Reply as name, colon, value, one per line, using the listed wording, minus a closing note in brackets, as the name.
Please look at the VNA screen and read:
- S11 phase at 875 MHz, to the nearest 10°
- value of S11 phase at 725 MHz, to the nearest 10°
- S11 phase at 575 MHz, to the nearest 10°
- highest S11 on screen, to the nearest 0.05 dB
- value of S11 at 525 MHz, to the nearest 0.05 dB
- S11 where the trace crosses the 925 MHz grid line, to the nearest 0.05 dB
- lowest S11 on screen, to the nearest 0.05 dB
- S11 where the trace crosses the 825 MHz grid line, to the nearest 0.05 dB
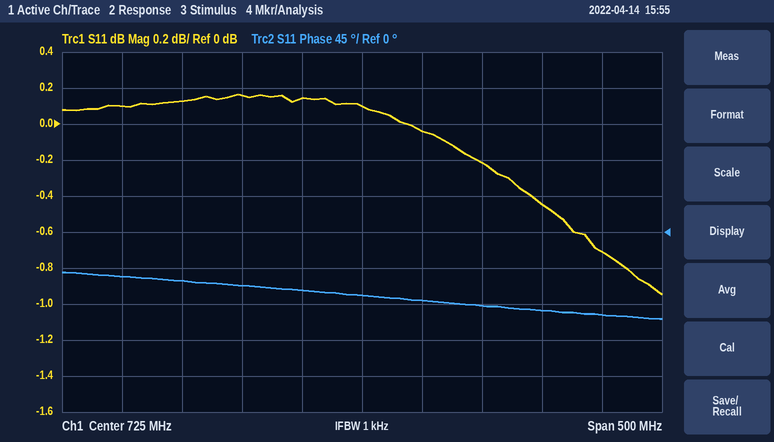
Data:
S11 phase at 875 MHz, to the nearest 10°: -100°
value of S11 phase at 725 MHz, to the nearest 10°: -80°
S11 phase at 575 MHz, to the nearest 10°: -60°
highest S11 on screen, to the nearest 0.05 dB: 0.15 dB
value of S11 at 525 MHz, to the nearest 0.05 dB: 0.10 dB
S11 where the trace crosses the 925 MHz grid line, to the nearest 0.05 dB: -0.70 dB
lowest S11 on screen, to the nearest 0.05 dB: -0.95 dB
S11 where the trace crosses the 825 MHz grid line, to the nearest 0.05 dB: -0.20 dB
